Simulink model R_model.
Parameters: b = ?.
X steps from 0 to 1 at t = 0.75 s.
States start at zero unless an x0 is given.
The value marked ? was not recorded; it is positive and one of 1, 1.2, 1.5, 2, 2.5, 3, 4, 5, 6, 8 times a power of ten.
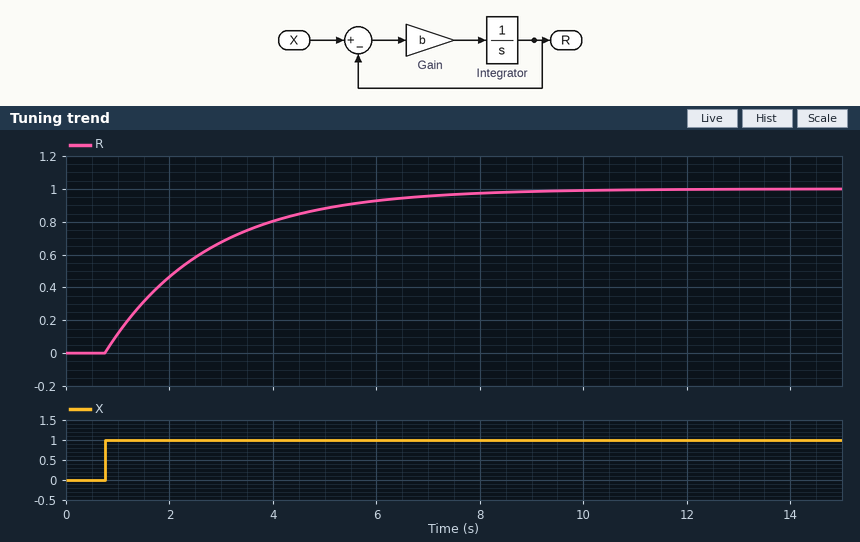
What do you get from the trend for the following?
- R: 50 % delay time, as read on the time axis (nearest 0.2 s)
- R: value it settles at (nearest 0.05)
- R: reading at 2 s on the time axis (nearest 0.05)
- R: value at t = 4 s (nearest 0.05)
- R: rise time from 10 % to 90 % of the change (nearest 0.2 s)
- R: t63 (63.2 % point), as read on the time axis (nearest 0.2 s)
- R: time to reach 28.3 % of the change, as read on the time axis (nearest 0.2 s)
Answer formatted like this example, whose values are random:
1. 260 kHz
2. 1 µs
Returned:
1. 2.2 s
2. 1.00
3. 0.45
4. 0.80
5. 4.4 s
6. 2.8 s
7. 1.4 s
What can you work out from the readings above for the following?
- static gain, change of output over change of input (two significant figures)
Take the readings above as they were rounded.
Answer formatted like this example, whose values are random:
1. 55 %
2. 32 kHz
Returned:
1. 1.0
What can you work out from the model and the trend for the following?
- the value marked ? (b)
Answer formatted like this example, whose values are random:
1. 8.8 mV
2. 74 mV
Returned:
1. 0.5
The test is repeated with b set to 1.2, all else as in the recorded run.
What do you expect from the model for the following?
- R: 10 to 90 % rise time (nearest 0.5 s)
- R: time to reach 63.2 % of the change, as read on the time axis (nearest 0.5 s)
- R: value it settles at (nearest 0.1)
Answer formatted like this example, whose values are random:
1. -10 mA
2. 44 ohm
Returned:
1. 2.0 s
2. 1.5 s
3. 1.0
